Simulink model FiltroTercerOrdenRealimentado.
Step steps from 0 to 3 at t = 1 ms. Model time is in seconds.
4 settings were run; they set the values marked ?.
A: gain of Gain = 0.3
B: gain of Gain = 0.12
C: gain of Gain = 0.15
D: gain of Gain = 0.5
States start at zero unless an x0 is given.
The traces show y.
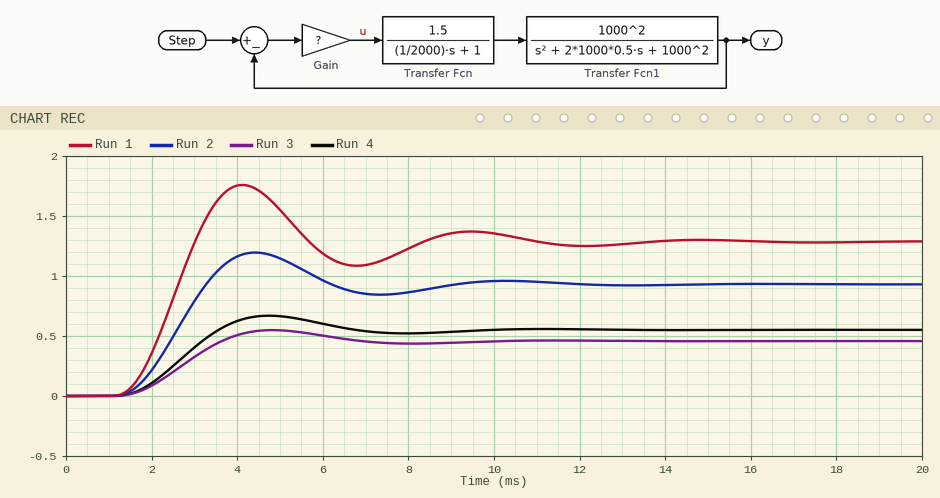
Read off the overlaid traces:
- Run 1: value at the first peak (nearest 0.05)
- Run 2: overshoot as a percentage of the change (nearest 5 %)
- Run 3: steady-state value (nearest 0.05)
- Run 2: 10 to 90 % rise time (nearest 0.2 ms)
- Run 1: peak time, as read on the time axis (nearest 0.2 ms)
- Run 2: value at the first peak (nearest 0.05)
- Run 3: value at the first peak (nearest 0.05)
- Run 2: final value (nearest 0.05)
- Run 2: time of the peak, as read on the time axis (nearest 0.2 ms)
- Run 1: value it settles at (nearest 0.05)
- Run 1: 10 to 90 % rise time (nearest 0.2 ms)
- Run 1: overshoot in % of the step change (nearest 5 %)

1.75
30 %
0.45
1.4 ms
4.2 ms
1.20
0.55
0.95
4.4 ms
1.30
1.2 ms
35 %
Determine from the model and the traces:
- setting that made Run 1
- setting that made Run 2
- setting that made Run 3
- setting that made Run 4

D
A
B
C
